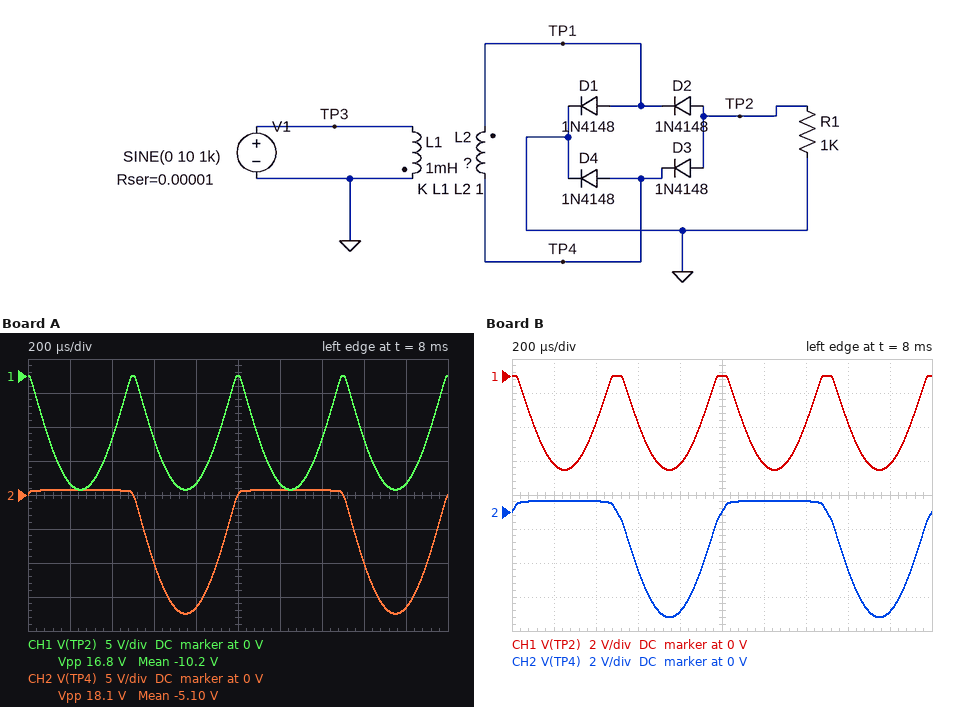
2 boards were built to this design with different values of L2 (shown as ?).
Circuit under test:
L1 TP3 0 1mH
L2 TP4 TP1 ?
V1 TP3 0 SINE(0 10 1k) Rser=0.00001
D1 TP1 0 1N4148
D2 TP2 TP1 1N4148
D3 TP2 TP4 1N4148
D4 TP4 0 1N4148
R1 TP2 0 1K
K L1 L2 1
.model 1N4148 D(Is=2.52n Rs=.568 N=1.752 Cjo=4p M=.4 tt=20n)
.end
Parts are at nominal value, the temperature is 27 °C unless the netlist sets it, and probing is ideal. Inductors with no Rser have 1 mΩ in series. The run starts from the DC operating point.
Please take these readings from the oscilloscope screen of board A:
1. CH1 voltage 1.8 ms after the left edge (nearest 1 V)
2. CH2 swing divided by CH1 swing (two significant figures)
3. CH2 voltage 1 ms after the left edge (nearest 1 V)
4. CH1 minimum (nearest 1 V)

-16 V
1.1
0 V
-17 V
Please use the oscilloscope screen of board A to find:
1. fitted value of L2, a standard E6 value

3.3 mH
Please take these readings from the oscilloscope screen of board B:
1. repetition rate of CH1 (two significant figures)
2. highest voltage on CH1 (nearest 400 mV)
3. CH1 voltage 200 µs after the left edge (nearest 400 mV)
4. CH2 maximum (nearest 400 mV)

2.0 kHz
0 V
-5.2 V
800 mV
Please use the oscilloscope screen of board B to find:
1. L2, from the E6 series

470 µH
